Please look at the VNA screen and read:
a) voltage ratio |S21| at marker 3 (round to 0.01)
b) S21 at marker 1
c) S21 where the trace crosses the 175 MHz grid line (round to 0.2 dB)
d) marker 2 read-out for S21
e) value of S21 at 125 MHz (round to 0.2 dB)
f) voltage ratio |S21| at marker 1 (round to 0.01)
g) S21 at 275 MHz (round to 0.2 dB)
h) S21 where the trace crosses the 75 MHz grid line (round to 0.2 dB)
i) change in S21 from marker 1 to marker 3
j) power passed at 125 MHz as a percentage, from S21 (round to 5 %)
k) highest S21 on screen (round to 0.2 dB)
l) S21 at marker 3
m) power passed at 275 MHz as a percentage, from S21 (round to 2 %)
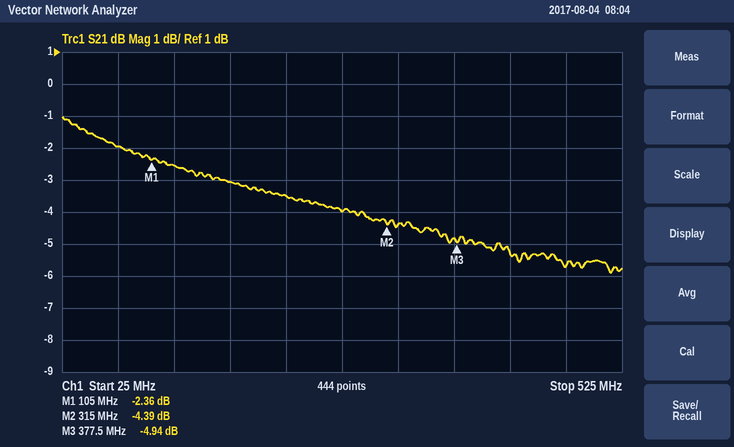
0.57
-2.36 dB
-3.0 dB
-4.39 dB
-2.6 dB
0.76
-4.0 dB
-2.0 dB
-2.58 dB
55 %
-1.0 dB
-4.94 dB
40 %
